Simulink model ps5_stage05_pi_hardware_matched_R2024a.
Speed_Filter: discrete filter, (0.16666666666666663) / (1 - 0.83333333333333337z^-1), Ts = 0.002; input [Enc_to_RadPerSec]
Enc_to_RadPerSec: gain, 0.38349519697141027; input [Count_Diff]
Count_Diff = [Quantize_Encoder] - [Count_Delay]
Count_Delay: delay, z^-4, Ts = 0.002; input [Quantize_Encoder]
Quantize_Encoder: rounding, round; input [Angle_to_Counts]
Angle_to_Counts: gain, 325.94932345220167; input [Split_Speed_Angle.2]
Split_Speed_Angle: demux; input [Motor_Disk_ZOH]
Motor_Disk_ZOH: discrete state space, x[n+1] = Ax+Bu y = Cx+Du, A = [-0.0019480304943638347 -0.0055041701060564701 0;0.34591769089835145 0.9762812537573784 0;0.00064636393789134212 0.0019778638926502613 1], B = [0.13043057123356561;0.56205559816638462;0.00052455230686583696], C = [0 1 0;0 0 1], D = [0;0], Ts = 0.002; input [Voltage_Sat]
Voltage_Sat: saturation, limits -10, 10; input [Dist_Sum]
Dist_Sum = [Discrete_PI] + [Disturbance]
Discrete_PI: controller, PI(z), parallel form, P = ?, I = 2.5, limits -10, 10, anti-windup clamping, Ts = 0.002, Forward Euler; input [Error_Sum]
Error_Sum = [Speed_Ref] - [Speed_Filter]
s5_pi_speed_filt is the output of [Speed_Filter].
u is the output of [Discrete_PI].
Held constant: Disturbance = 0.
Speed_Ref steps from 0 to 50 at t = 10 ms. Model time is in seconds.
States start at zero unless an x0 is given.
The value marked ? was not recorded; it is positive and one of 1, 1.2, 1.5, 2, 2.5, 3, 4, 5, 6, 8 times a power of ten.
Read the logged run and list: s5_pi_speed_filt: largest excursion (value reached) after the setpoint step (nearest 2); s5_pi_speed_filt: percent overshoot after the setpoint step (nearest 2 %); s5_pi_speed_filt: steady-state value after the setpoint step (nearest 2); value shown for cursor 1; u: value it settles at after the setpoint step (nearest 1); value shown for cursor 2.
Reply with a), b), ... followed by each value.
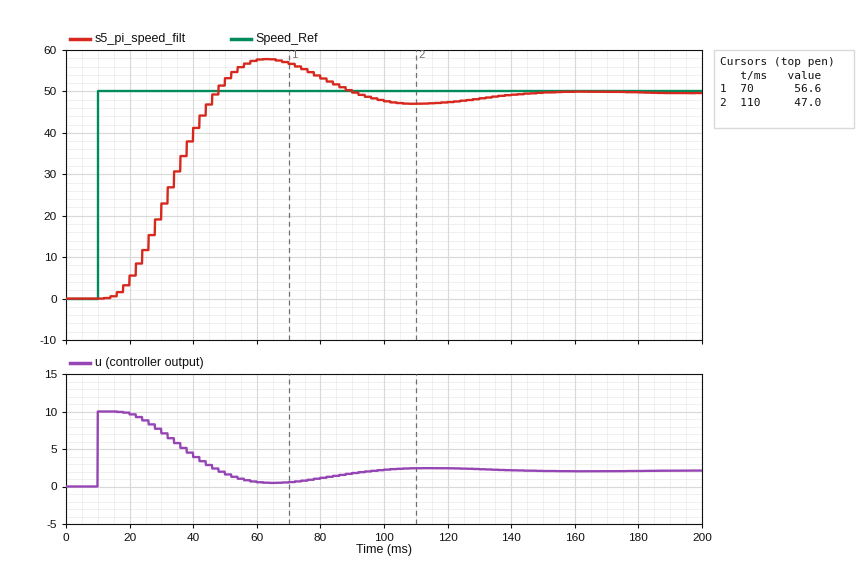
a) 58
b) 16 %
c) 50
d) 56.6
e) 2
f) 47.0
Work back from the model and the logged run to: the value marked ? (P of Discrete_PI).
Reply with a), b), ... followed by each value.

a) 0.2
